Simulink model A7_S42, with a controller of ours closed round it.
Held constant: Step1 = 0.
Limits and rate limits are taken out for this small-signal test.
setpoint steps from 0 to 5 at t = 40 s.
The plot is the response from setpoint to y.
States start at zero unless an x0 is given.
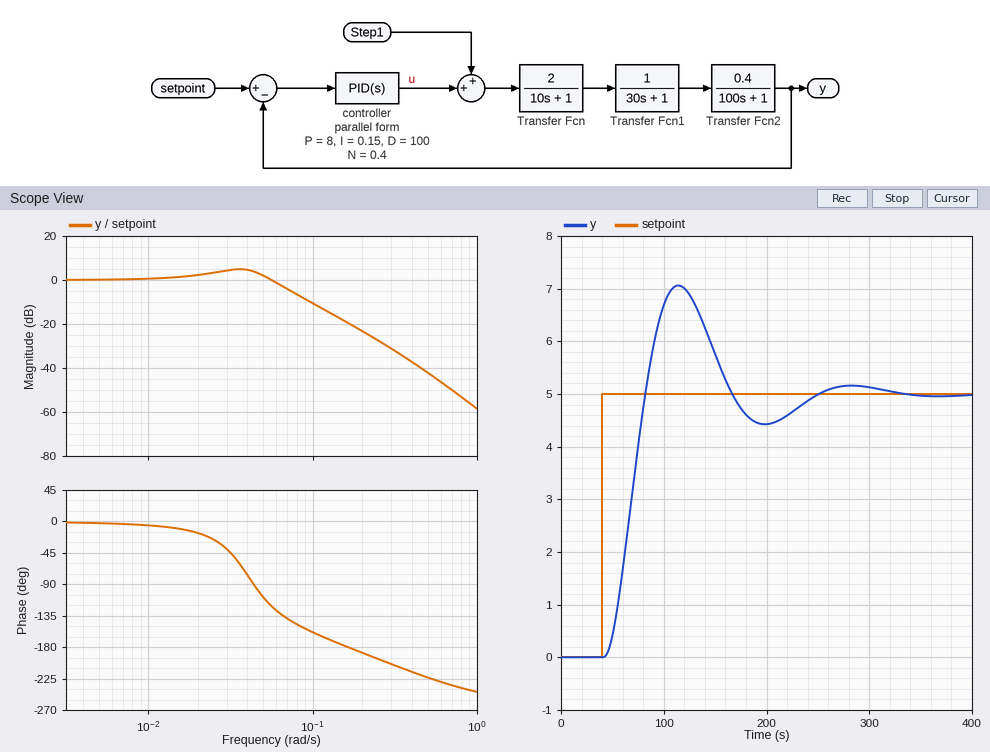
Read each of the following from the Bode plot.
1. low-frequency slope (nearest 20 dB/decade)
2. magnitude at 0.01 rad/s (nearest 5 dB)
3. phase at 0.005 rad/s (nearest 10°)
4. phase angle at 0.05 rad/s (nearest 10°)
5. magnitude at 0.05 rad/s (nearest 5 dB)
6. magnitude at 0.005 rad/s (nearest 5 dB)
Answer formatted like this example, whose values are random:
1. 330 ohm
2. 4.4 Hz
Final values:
1. 0 dB/decade
2. 0 dB
3. 0°
4. -110°
5. 0 dB
6. 0 dB
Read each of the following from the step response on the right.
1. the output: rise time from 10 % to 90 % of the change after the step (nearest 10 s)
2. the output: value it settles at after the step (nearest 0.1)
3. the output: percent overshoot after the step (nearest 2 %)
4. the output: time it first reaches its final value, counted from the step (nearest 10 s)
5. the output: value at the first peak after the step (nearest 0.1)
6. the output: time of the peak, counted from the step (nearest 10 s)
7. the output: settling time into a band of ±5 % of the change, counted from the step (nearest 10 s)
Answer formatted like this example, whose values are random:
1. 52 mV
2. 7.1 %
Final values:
1. 30 s
2. 5.0
3. 42 %
4. 40 s
5. 7.1
6. 70 s
7. 190 s
